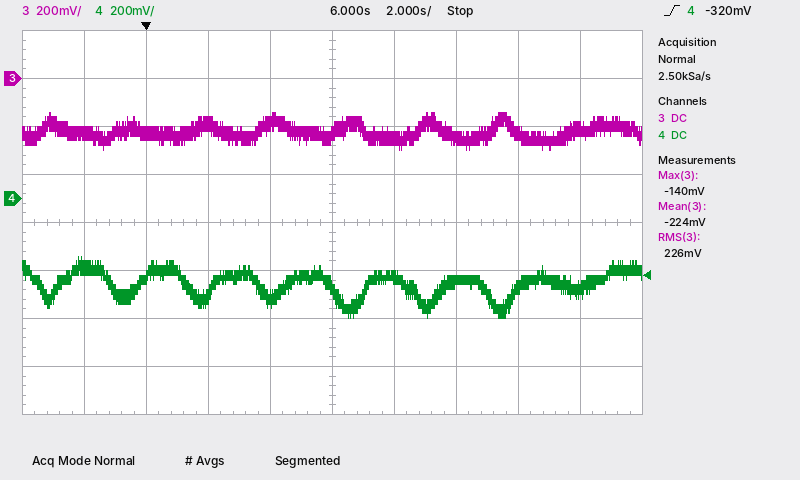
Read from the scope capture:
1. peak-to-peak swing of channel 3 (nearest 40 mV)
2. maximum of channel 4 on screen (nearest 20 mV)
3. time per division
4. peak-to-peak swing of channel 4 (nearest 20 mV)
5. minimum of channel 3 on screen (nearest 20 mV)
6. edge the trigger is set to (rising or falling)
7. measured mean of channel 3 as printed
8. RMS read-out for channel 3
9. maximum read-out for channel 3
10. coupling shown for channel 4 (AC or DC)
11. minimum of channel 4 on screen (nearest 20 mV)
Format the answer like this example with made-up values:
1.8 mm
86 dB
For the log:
160 mV
-240 mV
2 s
260 mV
-300 mV
rising
-224 mV
226 mV
-140 mV
DC
-500 mV
